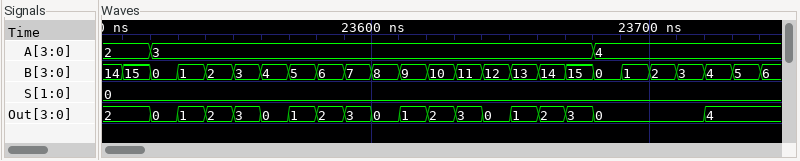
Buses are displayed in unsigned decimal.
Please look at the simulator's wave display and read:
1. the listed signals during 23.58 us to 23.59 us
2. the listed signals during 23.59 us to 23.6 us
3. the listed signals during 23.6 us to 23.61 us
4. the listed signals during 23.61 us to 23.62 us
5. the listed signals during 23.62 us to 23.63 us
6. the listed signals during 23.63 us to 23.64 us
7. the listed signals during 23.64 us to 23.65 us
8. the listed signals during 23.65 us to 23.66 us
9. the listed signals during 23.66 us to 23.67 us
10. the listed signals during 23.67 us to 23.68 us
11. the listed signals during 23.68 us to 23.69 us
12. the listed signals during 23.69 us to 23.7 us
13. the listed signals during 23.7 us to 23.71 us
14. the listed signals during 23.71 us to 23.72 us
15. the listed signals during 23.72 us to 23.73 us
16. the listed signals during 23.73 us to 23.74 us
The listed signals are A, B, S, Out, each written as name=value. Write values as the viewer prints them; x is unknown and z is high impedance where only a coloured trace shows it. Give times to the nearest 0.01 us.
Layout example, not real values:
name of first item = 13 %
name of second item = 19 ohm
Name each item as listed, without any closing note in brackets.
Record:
the listed signals during 23.58 us to 23.59 us = A=3, B=6, S=0, Out=2
the listed signals during 23.59 us to 23.6 us = A=3, B=7, S=0, Out=3
the listed signals during 23.6 us to 23.61 us = A=3, B=8, S=0, Out=0
the listed signals during 23.61 us to 23.62 us = A=3, B=9, S=0, Out=1
the listed signals during 23.62 us to 23.63 us = A=3, B=10, S=0, Out=2
the listed signals during 23.63 us to 23.64 us = A=3, B=11, S=0, Out=3
the listed signals during 23.64 us to 23.65 us = A=3, B=12, S=0, Out=0
the listed signals during 23.65 us to 23.66 us = A=3, B=13, S=0, Out=1
the listed signals during 23.66 us to 23.67 us = A=3, B=14, S=0, Out=2
the listed signals during 23.67 us to 23.68 us = A=3, B=15, S=0, Out=3
the listed signals during 23.68 us to 23.69 us = A=4, B=0, S=0, Out=0
the listed signals during 23.69 us to 23.7 us = A=4, B=1, S=0, Out=0
the listed signals during 23.7 us to 23.71 us = A=4, B=2, S=0, Out=0
the listed signals during 23.71 us to 23.72 us = A=4, B=3, S=0, Out=0
the listed signals during 23.72 us to 23.73 us = A=4, B=4, S=0, Out=4
the listed signals during 23.73 us to 23.74 us = A=4, B=5, S=0, Out=4
